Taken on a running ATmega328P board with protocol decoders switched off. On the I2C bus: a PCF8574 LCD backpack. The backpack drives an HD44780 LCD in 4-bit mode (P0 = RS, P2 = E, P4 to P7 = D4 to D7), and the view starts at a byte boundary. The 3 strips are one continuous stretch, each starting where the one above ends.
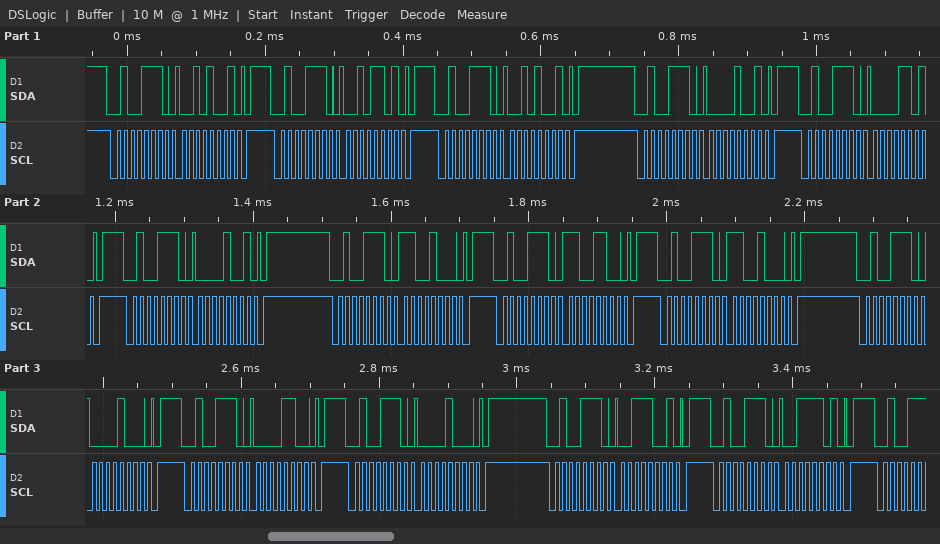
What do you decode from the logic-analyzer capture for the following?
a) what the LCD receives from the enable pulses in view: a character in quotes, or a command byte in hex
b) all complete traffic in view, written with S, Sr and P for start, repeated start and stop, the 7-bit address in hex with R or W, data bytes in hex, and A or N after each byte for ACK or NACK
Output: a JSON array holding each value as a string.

["' ' 0xC0", "S 27W A 29 A P S 27W A 2D A P S 27W A 29 A P S 27W A 09 A P S 27W A 0D A P S 27W A 09 A P S 27W A C8 A P S 27W A CC A P S 27W A C8 A P S 27W A 08 A P S 27W A 0C A P S 27W A 08 A P S 27W A 39 A P S 27W A 3D A P"]
